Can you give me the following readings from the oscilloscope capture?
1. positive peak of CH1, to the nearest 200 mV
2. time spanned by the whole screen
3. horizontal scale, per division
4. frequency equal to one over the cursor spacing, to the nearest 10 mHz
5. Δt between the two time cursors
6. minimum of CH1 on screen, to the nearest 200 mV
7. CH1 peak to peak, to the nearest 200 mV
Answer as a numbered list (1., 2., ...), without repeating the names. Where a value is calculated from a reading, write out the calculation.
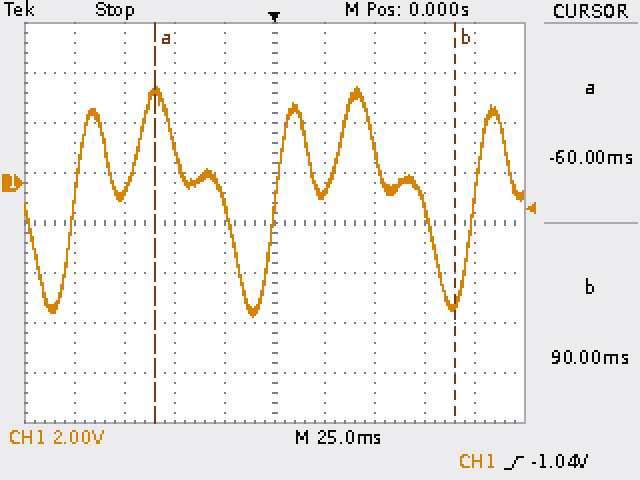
1. 3.8 V
2. 250 ms
3. 25 ms
4. 1 / 150.0 ms ≈ 6.67 Hz
5. 90 ms − (-60 ms) = 150.0 ms
6. -5.4 V
7. 3.8 V − (-5.4 V) = 9.2 V
